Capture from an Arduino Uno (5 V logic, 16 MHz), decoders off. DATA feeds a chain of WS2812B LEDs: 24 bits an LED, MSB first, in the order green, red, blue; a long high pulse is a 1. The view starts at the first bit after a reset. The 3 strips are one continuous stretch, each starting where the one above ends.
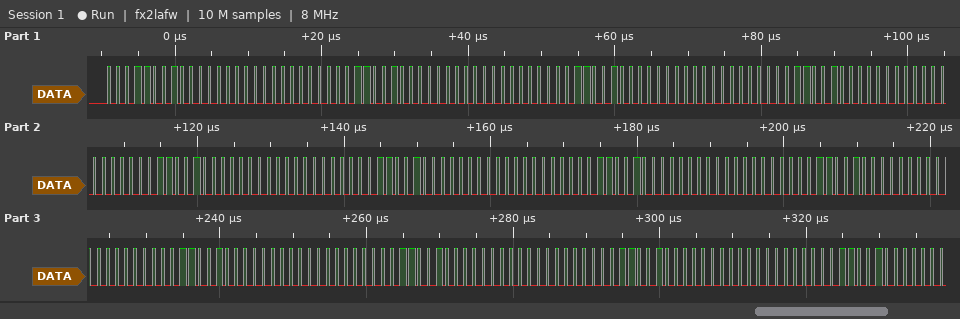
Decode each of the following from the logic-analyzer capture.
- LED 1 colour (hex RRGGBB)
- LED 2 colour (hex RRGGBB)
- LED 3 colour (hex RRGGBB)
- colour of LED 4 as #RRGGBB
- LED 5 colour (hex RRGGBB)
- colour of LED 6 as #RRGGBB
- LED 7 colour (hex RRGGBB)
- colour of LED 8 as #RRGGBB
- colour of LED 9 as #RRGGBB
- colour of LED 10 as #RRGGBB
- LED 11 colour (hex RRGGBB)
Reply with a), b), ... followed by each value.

a) #001900
b) #001900
c) #001900
d) #001900
e) #001900
f) #001900
g) #001900
h) #001900
i) #001900
j) #001900
k) #001900
